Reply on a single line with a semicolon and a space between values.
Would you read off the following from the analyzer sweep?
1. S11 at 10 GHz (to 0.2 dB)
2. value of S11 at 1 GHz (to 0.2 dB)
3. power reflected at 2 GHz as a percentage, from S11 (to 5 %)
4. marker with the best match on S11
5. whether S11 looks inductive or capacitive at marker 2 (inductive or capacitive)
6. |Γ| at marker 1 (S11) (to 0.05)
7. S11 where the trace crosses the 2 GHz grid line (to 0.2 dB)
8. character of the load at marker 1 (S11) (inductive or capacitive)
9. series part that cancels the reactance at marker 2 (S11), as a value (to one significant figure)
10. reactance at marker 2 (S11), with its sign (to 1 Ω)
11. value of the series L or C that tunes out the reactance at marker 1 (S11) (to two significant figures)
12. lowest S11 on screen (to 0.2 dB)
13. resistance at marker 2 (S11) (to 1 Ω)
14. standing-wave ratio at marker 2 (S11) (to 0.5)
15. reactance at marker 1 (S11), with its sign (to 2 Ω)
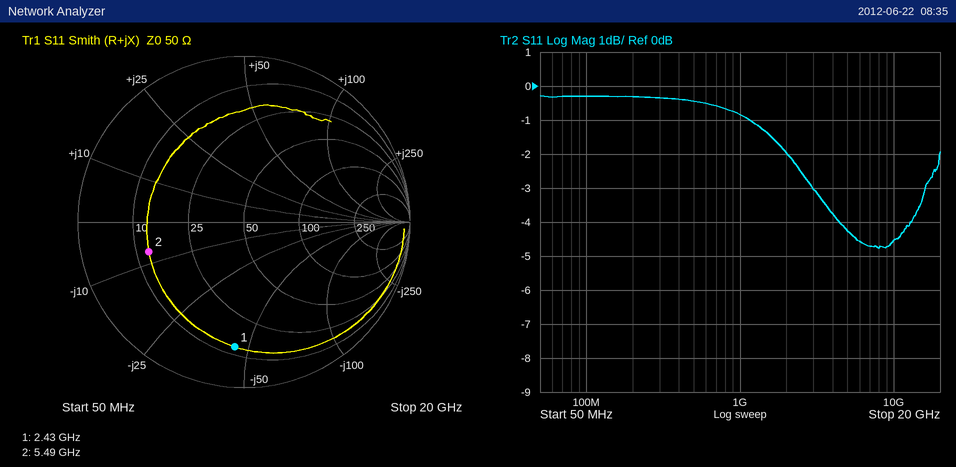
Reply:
-4.6 dB; -0.8 dB; 65 %; marker 2; capacitive; 0.75; -2.0 dB; capacitive; 200 pH; -7 Ω; 2.9 nH; -4.8 dB; 13 Ω; 4.0; -44 Ω
